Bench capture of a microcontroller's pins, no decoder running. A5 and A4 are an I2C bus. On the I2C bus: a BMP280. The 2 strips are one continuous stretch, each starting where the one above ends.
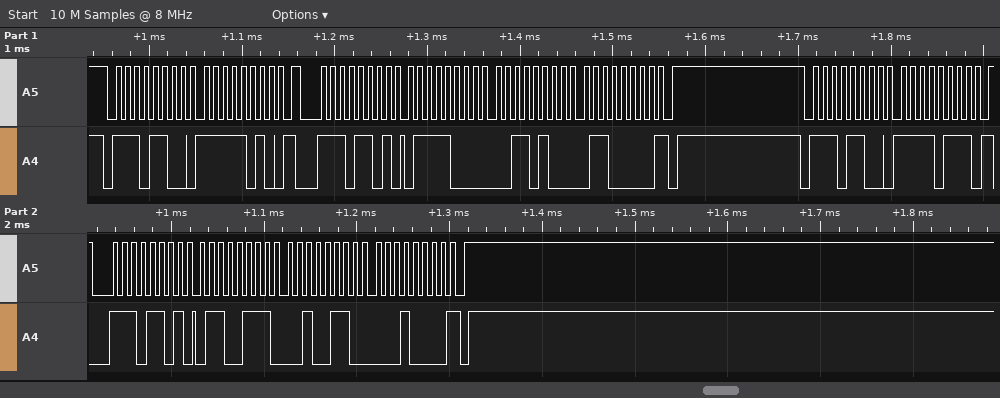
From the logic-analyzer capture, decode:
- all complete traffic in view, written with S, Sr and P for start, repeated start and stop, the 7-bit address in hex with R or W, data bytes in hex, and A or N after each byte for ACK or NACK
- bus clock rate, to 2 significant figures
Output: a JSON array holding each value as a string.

["S 76W A FA A Sr 76R A 78 A 34 A 60 N P S 76W A F7 A Sr 76R A 67 A 26 A 10 N P", "100 kHz"]
